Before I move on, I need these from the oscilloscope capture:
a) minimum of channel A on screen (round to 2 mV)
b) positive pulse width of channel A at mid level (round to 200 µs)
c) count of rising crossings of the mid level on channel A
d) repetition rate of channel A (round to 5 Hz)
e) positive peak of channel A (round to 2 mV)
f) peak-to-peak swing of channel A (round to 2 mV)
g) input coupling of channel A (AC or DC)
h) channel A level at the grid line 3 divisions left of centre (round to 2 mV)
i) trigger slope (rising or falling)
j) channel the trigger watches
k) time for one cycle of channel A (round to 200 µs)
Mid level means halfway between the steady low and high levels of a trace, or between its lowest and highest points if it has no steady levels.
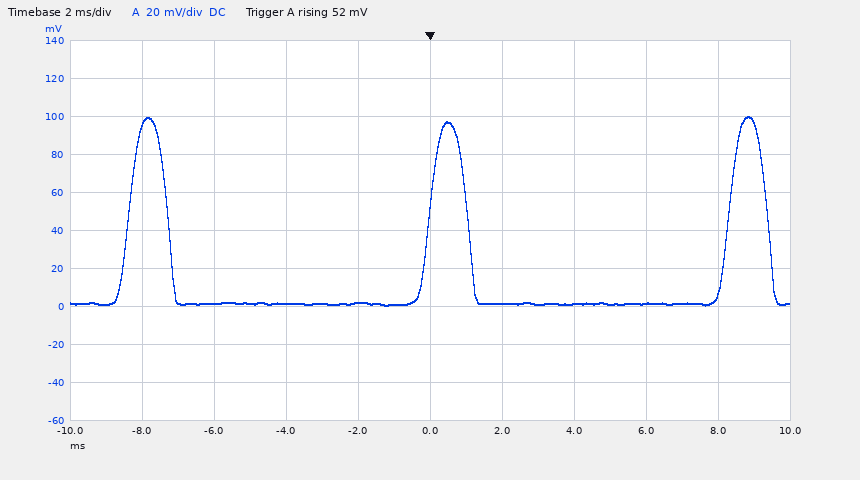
0 mV
1.0 ms
3
120 Hz
100 mV
100 mV
DC
2 mV
rising
channel A
8.4 ms
